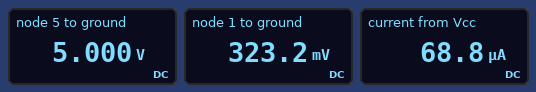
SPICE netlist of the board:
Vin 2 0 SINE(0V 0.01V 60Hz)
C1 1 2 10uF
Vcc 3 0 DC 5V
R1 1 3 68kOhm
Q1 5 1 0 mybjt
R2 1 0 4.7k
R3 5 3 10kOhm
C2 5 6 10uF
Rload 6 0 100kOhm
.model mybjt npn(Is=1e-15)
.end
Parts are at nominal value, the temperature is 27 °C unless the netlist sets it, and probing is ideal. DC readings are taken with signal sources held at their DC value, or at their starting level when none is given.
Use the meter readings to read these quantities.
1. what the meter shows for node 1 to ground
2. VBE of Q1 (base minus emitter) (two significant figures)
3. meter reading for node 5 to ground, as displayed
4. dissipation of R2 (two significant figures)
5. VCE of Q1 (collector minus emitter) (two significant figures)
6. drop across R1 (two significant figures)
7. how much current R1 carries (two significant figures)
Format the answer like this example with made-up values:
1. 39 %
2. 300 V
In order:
1. 323.2 mV
2. 320 mV
3. 5.000 V
4. 22 µW
5. 5.0 V
6. 4.7 V
7. 69 µA
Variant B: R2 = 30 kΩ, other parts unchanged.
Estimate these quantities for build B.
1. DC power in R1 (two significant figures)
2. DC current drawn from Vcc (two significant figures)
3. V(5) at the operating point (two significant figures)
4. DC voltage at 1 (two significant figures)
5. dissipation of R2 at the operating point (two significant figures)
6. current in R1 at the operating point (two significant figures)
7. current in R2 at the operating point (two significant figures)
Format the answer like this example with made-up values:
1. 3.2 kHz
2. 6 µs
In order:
1. 270 µW
2. 560 µA
3. 72 mV
4. 700 mV
5. 16 µW
6. 63 µA
7. 23 µA
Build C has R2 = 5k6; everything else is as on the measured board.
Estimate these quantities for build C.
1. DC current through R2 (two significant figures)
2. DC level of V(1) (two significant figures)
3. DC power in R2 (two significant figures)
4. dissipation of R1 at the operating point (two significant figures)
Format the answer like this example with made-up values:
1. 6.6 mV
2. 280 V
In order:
1. 68 µA
2. 380 mV
3. 26 µW
4. 310 µW
